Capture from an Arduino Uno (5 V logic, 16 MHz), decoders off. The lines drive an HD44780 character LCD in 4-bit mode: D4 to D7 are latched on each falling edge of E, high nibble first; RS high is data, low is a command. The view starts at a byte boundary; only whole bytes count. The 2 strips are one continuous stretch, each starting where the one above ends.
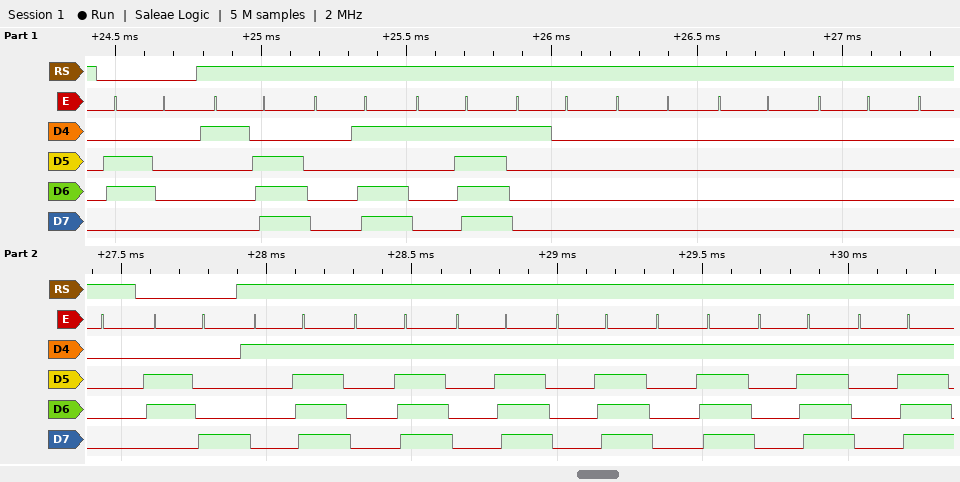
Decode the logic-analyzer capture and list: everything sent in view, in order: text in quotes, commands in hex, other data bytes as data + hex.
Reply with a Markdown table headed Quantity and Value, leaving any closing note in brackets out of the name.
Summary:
| Quantity | Value |
|---|---|
| everything sent in view, in order: text in quotes, commands in hex, other data bytes as data + hex | 0x60 data 1E 0D 1F 10 00 00 00 00 0x68 data 1F 1F 1F 1F 1F 1F 1F |
